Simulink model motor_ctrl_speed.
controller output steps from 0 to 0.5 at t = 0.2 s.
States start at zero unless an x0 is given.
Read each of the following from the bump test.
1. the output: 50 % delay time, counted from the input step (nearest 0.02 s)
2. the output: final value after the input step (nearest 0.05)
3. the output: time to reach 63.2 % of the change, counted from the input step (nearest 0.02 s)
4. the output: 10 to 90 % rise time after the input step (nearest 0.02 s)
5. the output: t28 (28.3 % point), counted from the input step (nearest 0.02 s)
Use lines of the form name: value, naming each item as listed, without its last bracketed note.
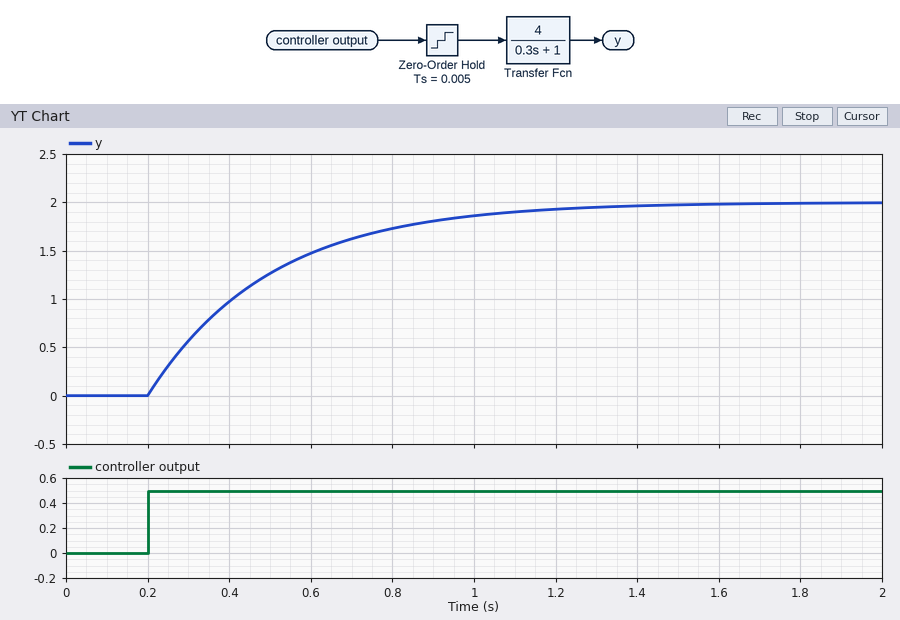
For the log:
the output: 50 % delay time, counted from the input step: 0.20 s
the output: final value after the input step: 2.00
the output: time to reach 63.2 % of the change, counted from the input step: 0.30 s
the output: 10 to 90 % rise time after the input step: 0.66 s
the output: t28 (28.3 % point), counted from the input step: 0.10 s
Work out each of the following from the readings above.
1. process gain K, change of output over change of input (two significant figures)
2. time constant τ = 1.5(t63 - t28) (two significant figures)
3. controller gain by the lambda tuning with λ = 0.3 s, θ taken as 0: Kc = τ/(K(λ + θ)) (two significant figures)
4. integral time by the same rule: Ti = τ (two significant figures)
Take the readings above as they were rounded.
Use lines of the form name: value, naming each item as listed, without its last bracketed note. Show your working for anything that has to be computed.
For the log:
process gain K, change of output over change of input: (2 - 0) / 0.5 = 4.0
time constant τ = 1.5(t63 - t28): 1.5 × (0.3 - 0.1) = 0.30 s
controller gain by the lambda tuning with λ = 0.3 s, θ taken as 0: Kc = τ/(K(λ + θ)): 0.3 / (4 × (0.3 + 0)) = 0.25
integral time by the same rule: Ti = τ: 0.30 s
